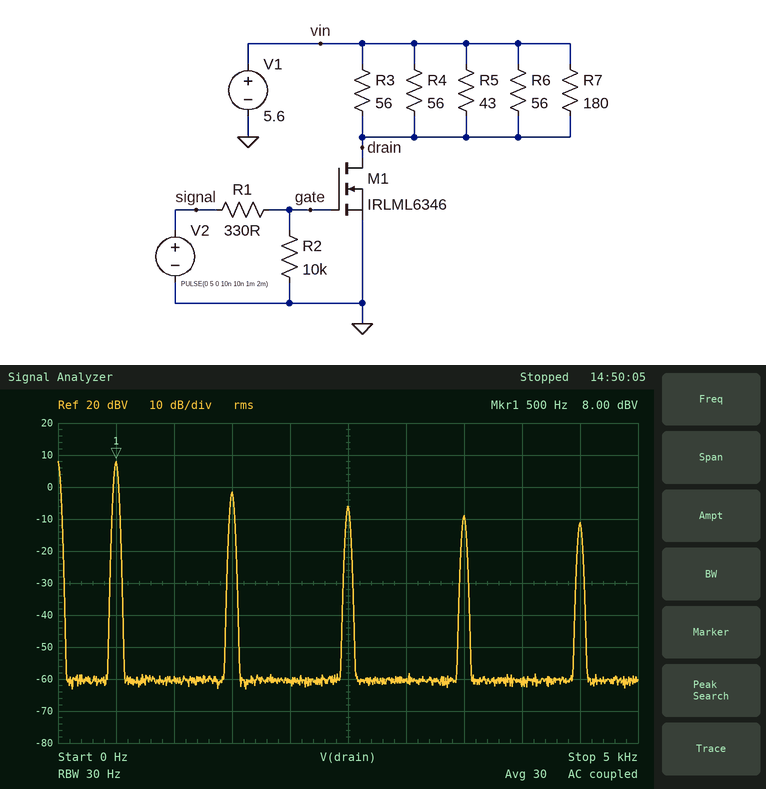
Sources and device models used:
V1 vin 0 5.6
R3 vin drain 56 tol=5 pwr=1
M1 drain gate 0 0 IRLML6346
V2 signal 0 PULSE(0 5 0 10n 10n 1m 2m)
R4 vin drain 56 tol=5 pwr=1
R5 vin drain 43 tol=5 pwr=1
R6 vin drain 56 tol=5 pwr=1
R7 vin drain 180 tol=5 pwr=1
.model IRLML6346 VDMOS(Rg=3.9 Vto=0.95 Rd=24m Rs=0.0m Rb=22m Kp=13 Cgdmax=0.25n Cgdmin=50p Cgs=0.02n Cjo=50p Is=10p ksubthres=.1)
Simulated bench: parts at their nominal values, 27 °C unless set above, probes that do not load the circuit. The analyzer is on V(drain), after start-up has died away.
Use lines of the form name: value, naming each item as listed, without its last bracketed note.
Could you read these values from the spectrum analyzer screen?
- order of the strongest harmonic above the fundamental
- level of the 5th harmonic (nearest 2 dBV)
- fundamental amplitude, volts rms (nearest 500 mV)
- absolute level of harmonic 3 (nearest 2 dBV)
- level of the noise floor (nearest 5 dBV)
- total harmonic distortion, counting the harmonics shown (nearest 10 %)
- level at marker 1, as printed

order of the strongest harmonic above the fundamental: 3
level of the 5th harmonic: -6 dBV
fundamental amplitude, volts rms: 2.5 V
absolute level of harmonic 3: -2 dBV
level of the noise floor: -60 dBV
total harmonic distortion, counting the harmonics shown: 40 %
level at marker 1, as printed: 8.00 dBV
